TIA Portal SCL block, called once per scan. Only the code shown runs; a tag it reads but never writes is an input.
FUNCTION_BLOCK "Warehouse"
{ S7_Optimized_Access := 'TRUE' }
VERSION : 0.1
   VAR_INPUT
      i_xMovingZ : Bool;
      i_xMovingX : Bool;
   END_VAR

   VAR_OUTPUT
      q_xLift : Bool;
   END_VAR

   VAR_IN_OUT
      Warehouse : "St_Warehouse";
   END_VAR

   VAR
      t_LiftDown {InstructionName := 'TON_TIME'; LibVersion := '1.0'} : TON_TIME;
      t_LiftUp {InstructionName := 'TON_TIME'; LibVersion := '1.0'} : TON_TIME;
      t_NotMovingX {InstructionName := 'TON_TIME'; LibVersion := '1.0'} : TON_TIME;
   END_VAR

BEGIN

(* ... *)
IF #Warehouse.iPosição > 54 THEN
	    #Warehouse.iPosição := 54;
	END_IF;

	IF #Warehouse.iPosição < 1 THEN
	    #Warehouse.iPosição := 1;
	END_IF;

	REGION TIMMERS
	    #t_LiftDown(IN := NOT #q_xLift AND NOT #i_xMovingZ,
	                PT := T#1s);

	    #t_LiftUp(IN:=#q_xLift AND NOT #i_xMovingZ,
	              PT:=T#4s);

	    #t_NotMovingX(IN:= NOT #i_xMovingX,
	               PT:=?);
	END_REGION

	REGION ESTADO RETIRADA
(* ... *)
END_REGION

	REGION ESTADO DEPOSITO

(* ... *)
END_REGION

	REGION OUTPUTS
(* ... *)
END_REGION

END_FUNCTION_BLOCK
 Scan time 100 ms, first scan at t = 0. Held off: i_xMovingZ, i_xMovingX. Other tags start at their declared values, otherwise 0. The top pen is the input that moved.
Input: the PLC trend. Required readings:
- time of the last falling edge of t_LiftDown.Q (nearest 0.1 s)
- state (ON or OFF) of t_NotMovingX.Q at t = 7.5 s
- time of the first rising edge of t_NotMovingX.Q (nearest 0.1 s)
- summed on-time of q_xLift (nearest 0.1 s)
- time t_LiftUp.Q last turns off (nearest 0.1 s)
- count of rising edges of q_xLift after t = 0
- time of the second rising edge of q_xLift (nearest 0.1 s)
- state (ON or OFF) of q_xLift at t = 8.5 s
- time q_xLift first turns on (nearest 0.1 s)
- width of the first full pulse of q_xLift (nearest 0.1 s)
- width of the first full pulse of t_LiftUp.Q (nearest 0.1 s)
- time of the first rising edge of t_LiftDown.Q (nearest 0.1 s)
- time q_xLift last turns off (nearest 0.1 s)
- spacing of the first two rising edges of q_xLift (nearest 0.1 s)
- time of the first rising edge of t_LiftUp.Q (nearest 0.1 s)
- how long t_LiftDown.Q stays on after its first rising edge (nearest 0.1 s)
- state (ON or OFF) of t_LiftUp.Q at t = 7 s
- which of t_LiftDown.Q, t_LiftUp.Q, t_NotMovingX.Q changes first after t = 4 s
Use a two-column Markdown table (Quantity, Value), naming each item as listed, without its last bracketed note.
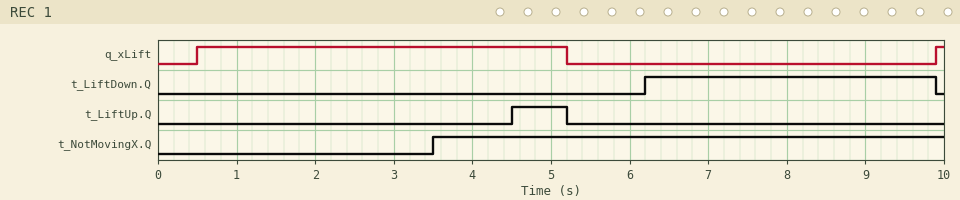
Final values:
| Quantity | Value |
|---|---|
| time of the last falling edge of t_LiftDown.Q | 9.9 s |
| state (ON or OFF) of t_NotMovingX.Q at t = 7.5 s | ON |
| time of the first rising edge of t_NotMovingX.Q | 3.5 s |
| summed on-time of q_xLift | 4.8 s |
| time t_LiftUp.Q last turns off | 5.2 s |
| count of rising edges of q_xLift after t = 0 | 2 |
| time of the second rising edge of q_xLift | 9.9 s |
| state (ON or OFF) of q_xLift at t = 8.5 s | OFF |
| time q_xLift first turns on | 0.5 s |
| width of the first full pulse of q_xLift | 4.7 s |
| width of the first full pulse of t_LiftUp.Q | 0.7 s |
| time of the first rising edge of t_LiftDown.Q | 6.2 s |
| time q_xLift last turns off | 5.2 s |
| spacing of the first two rising edges of q_xLift | 9.4 s |
| time of the first rising edge of t_LiftUp.Q | 4.5 s |
| how long t_LiftDown.Q stays on after its first rising edge | 3.7 s |
| state (ON or OFF) of t_LiftUp.Q at t = 7 s | OFF |
| which of t_LiftDown.Q, t_LiftUp.Q, t_NotMovingX.Q changes first after t = 4 s | t_LiftUp.Q |
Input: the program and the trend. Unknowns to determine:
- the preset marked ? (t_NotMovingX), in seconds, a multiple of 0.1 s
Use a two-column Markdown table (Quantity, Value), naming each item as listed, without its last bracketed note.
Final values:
| Quantity | Value |
|---|---|
| the preset marked ? (t_NotMovingX), in seconds, a multiple of 0.1 s | 3.5 s |
